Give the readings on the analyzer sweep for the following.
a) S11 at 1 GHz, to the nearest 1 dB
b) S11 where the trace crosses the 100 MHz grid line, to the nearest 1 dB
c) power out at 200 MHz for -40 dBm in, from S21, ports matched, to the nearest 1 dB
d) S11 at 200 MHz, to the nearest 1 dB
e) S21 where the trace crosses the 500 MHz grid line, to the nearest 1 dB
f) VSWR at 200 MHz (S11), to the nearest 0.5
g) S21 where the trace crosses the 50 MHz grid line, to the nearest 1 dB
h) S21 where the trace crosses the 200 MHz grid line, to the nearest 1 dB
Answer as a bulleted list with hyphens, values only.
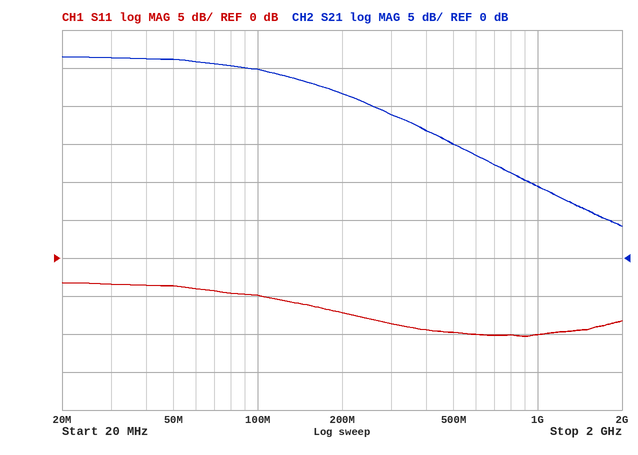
- -10 dB
- -5 dB
- -18 dBm
- -7 dB
- 15 dB
- 2.5
- 26 dB
- 22 dB
